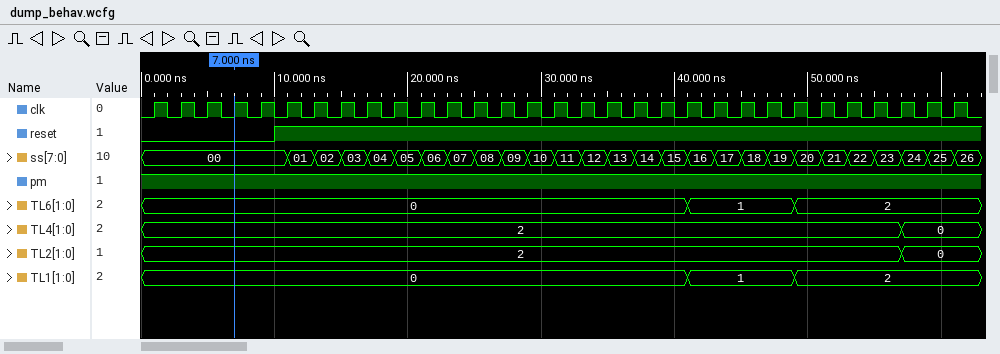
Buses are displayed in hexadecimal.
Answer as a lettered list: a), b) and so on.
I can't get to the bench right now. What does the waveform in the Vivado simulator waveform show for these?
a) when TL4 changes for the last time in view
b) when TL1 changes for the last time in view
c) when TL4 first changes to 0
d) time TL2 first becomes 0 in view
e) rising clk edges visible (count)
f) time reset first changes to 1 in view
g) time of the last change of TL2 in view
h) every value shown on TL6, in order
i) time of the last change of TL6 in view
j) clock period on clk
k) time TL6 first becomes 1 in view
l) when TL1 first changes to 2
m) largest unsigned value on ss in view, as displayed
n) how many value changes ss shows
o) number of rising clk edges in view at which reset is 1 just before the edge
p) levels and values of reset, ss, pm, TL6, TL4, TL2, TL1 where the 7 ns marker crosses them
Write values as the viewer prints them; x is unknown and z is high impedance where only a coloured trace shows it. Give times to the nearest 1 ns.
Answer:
a) 57 ns
b) 49 ns
c) 57 ns
d) 57 ns
e) 31
f) 10 ns
g) 57 ns
h) 0, 1, 2
i) 49 ns
j) 2 ns
k) 41 ns
l) 49 ns
m) 26
n) 26
o) 26
p) reset=0, ss=00, pm=1, TL6=0, TL4=2, TL2=2, TL1=0
